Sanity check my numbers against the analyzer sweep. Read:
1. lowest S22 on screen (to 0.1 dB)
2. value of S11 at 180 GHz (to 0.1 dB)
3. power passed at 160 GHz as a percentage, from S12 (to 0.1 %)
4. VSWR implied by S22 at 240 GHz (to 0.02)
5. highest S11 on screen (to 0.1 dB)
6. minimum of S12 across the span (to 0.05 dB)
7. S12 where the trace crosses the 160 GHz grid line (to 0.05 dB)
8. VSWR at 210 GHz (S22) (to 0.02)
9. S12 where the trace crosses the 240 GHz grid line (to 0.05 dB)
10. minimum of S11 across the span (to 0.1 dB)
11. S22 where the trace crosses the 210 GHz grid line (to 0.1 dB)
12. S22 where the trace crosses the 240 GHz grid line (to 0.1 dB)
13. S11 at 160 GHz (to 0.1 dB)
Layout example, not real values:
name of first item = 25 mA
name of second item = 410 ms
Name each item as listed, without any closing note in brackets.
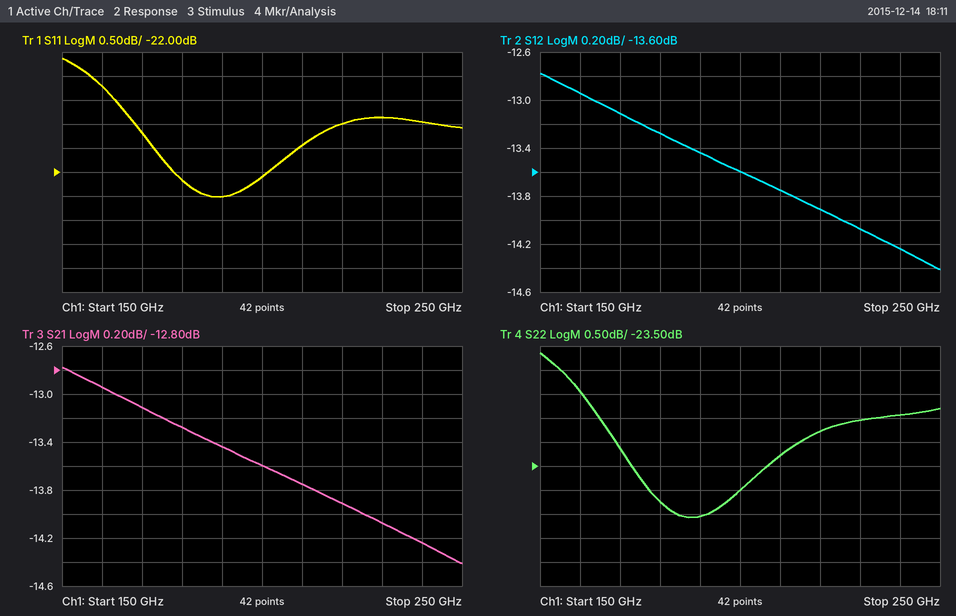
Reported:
lowest S22 on screen = -24.6 dB
value of S11 at 180 GHz = -22.2 dB
power passed at 160 GHz as a percentage, from S12 = 5.1 %
VSWR implied by S22 at 240 GHz = 1.16
highest S11 on screen = -19.6 dB
minimum of S12 across the span = -14.40 dB
S12 where the trace crosses the 160 GHz grid line = -12.95 dB
VSWR at 210 GHz (S22) = 1.14
S12 where the trace crosses the 240 GHz grid line = -14.25 dB
minimum of S11 across the span = -22.5 dB
S22 where the trace crosses the 210 GHz grid line = -23.3 dB
S22 where the trace crosses the 240 GHz grid line = -22.4 dB
S11 at 160 GHz = -20.2 dB
